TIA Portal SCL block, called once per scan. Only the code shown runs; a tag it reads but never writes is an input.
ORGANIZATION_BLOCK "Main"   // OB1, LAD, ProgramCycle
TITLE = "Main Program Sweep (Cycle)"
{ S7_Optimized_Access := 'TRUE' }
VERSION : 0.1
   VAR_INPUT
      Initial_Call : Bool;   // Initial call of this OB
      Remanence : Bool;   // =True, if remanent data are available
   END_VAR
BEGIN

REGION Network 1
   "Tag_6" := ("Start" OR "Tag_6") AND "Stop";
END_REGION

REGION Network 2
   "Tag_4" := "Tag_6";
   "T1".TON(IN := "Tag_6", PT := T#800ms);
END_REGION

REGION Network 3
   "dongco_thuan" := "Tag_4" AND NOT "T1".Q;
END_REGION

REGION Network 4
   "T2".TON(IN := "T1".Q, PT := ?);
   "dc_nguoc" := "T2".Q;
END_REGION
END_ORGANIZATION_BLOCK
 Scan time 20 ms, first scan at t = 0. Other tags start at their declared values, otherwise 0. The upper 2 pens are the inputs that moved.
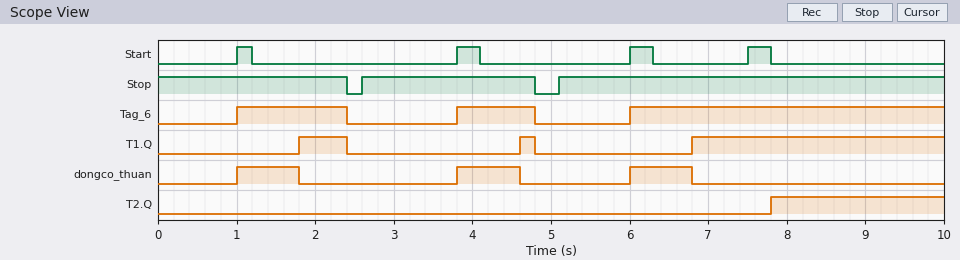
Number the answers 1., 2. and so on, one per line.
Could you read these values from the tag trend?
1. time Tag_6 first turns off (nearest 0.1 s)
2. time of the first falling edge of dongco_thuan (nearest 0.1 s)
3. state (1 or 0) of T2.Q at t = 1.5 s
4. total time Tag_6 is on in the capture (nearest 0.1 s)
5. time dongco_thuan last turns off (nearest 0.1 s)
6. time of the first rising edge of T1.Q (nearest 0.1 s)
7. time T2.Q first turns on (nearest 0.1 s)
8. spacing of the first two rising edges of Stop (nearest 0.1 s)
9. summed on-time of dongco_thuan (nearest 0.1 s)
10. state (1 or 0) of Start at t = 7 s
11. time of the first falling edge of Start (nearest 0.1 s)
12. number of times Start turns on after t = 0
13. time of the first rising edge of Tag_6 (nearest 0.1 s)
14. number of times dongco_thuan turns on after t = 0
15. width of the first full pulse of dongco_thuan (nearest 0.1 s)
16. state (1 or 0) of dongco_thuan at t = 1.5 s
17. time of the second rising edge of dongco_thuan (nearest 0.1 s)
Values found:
1. 2.4 s
2. 1.8 s
3. 0
4. 6.4 s
5. 6.8 s
6. 1.8 s
7. 7.8 s
8. 2.5 s
9. 2.4 s
10. 0
11. 1.2 s
12. 4
13. 1.0 s
14. 3
15. 0.8 s
16. 1
17. 3.8 s
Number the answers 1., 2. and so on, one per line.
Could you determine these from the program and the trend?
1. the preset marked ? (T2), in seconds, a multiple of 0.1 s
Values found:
1. 1.0 s
